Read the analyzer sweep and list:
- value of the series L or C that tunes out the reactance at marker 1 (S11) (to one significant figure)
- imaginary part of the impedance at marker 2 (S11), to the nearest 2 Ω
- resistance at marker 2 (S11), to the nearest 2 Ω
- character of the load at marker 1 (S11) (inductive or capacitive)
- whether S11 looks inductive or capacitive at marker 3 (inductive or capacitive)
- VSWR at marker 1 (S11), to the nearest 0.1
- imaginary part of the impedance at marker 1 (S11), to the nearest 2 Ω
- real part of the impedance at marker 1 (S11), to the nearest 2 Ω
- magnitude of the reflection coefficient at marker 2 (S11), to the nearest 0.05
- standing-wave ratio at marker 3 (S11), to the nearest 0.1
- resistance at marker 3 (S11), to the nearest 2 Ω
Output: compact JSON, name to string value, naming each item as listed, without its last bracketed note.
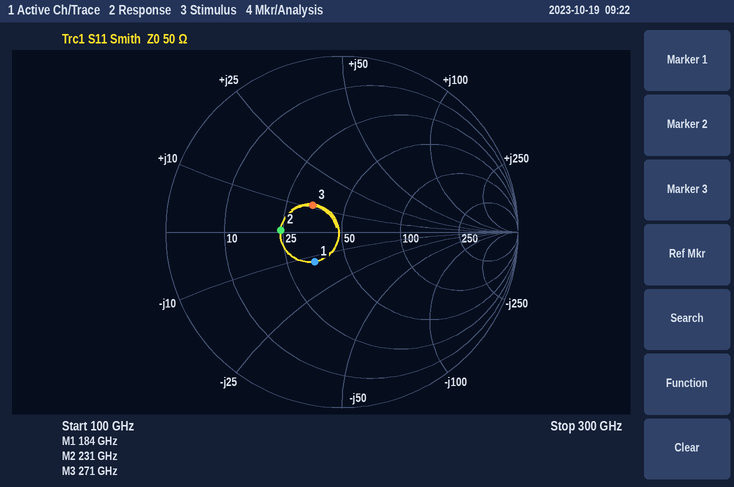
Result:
{"value of the series L or C that tunes out the reactance at marker 1 (S11)": "10 pH", "imaginary part of the impedance at marker 2 (S11), to the nearest 2 Ω": "0 Ω", "resistance at marker 2 (S11), to the nearest 2 Ω": "24 Ω", "character of the load at marker 1 (S11)": "capacitive", "whether S11 looks inductive or capacitive at marker 3": "inductive", "VSWR at marker 1 (S11), to the nearest 0.1": "1.6", "imaginary part of the impedance at marker 1 (S11), to the nearest 2 Ω": "-12 Ω", "real part of the impedance at marker 1 (S11), to the nearest 2 Ω": "34 Ω", "magnitude of the reflection coefficient at marker 2 (S11), to the nearest 0.05": "0.35", "standing-wave ratio at marker 3 (S11), to the nearest 0.1": "1.6", "resistance at marker 3 (S11), to the nearest 2 Ω": "34 Ω"}
